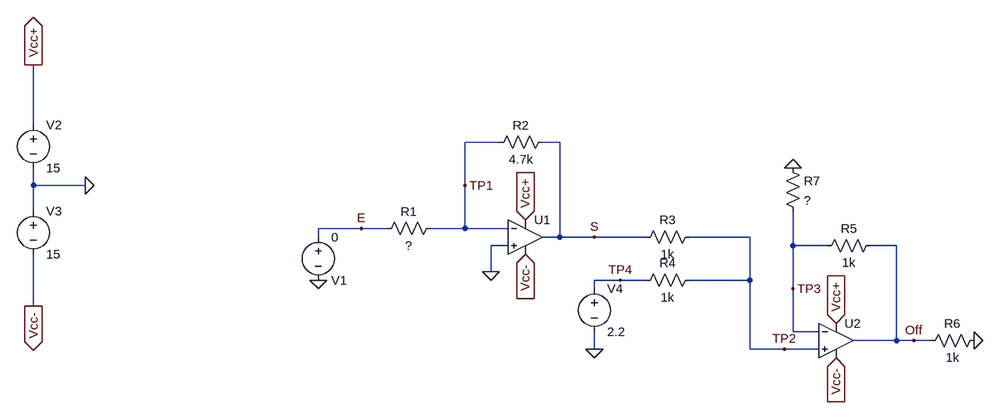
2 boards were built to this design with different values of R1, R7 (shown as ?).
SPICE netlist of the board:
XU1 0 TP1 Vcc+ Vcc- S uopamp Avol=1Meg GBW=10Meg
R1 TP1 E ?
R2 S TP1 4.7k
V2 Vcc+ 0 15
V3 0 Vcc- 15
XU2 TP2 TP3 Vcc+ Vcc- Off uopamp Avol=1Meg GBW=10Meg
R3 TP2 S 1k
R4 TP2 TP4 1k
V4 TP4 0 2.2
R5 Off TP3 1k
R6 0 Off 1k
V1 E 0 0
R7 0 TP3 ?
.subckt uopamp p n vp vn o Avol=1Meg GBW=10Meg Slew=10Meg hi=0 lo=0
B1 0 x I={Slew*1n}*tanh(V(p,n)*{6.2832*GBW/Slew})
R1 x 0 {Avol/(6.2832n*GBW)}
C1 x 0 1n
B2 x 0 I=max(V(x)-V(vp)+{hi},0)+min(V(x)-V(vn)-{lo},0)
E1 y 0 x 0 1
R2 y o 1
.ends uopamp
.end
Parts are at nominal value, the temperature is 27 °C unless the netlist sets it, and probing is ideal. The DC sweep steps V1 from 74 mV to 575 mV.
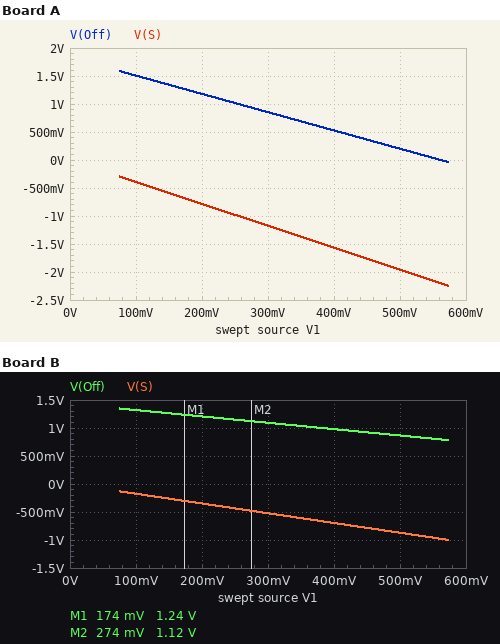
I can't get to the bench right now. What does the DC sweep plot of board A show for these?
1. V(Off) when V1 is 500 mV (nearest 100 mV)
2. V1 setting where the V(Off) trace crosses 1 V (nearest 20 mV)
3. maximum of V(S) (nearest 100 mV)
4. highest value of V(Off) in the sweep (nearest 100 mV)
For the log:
200 mV
260 mV
-300 mV
1.6 V
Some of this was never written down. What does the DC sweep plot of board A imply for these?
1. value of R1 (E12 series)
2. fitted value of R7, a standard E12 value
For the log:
1.2 kΩ
1.5 kΩ
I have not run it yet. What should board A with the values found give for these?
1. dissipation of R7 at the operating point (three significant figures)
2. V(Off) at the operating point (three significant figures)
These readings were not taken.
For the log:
807 µW
1.83 V
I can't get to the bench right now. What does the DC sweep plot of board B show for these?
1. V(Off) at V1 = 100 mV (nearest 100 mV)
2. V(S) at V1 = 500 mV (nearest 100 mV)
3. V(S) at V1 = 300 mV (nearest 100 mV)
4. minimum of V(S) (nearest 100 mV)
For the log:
1.3 V
-900 mV
-500 mV
-1.0 V
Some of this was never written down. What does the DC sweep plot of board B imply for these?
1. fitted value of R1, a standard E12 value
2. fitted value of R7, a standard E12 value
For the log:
2.7 kΩ
3.3 kΩ
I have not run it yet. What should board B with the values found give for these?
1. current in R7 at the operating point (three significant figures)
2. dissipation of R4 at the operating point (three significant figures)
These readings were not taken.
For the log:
333 µA
1.21 mW
